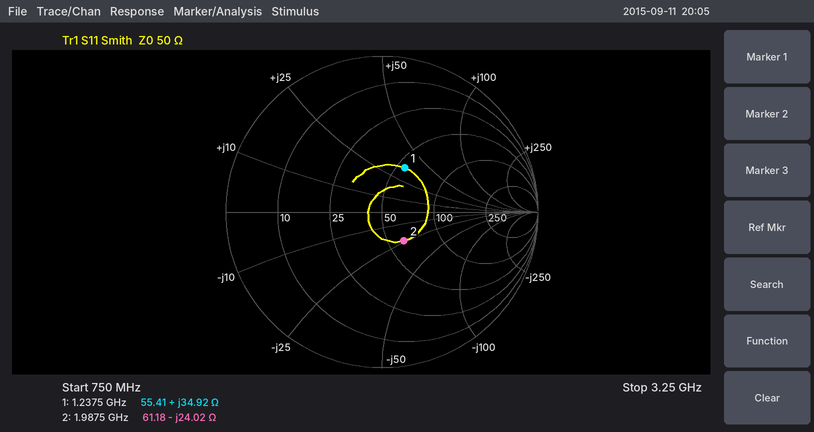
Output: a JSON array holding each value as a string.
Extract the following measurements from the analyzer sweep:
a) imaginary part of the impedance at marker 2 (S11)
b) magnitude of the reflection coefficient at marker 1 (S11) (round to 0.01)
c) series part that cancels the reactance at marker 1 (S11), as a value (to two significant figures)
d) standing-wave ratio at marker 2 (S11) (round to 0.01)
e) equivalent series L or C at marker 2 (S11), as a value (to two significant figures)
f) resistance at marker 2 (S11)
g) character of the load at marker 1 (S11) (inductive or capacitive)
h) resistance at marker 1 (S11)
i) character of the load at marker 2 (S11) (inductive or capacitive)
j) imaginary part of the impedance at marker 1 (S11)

["-24.02 Ω", "0.32", "3.7 pF", "1.61", "3.3 pF", "61.18 Ω", "inductive", "55.41 Ω", "capacitive", "+34.92 Ω"]
